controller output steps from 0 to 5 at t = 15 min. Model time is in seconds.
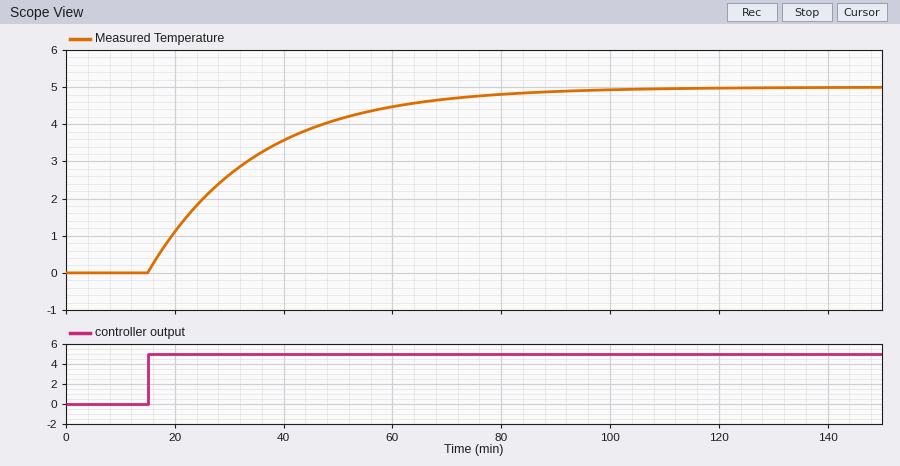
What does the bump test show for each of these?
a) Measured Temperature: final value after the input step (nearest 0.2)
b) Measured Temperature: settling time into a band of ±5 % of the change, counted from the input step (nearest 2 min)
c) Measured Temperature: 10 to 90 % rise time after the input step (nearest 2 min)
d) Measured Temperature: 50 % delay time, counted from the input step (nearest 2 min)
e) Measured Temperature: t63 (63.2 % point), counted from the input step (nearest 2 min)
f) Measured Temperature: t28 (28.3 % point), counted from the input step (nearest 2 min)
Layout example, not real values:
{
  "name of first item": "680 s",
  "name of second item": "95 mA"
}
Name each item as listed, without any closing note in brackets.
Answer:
{
  "Measured Temperature: final value after the input step": "5.0",
  "Measured Temperature: settling time into a band of ±5 % of the change, counted from the input step": "60 min",
  "Measured Temperature: 10 to 90 % rise time after the input step": "44 min",
  "Measured Temperature: 50 % delay time, counted from the input step": "14 min",
  "Measured Temperature: t63 (63.2 % point), counted from the input step": "20 min",
  "Measured Temperature: t28 (28.3 % point), counted from the input step": "6 min"
}
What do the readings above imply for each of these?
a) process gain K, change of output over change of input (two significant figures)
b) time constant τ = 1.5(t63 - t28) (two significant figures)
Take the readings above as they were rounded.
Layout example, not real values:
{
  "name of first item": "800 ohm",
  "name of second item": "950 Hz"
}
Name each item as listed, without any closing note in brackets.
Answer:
{
  "process gain K, change of output over change of input": "1.0",
  "time constant τ = 1.5(t63 - t28)": "21 min"
}
